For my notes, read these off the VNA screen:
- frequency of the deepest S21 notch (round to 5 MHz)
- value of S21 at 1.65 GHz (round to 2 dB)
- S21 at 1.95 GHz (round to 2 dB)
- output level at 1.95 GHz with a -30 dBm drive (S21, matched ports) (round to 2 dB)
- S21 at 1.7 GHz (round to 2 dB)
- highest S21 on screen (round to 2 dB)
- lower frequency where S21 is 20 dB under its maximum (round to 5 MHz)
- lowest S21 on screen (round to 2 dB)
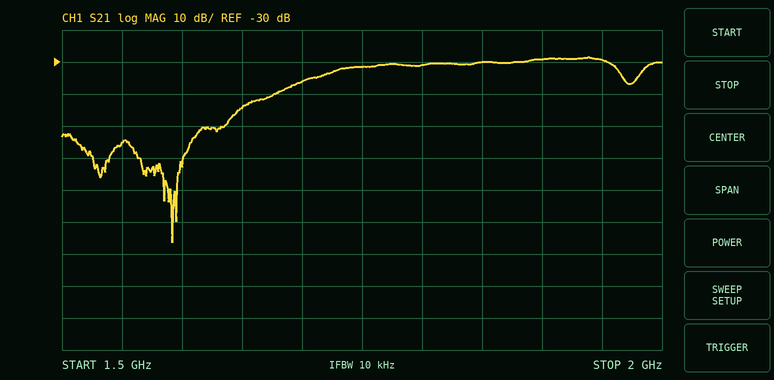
1.590 GHz
-44 dB
-30 dB
-60 dBm
-36 dB
-28 dB
1.640 GHz
-86 dB
